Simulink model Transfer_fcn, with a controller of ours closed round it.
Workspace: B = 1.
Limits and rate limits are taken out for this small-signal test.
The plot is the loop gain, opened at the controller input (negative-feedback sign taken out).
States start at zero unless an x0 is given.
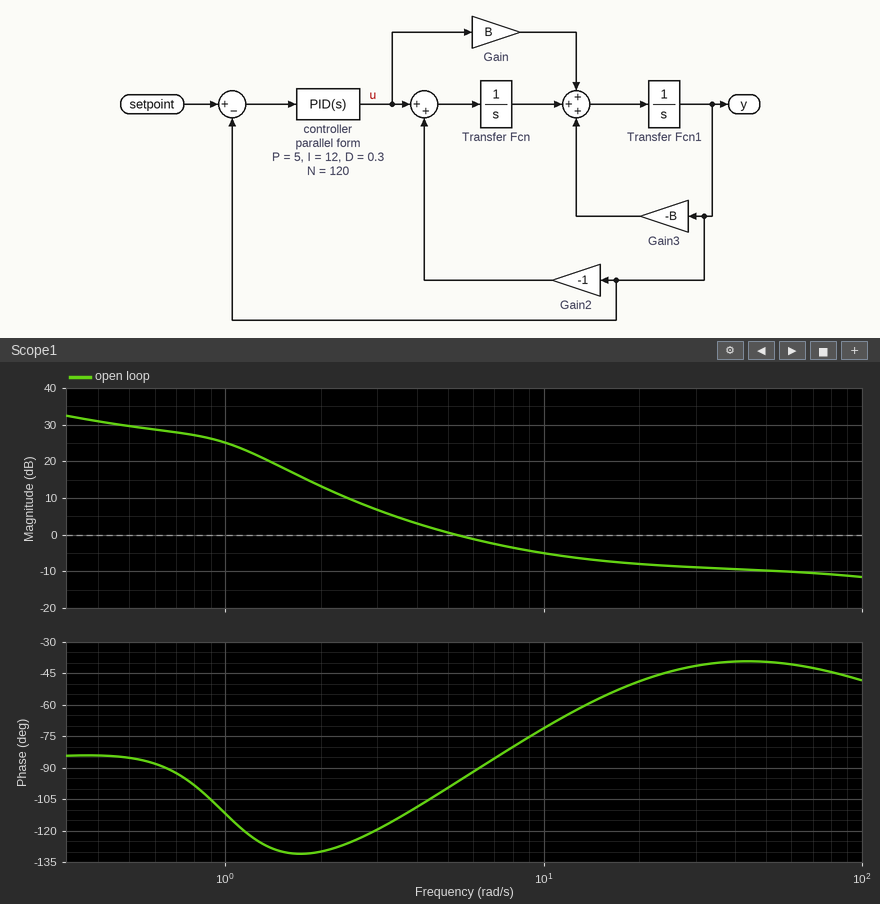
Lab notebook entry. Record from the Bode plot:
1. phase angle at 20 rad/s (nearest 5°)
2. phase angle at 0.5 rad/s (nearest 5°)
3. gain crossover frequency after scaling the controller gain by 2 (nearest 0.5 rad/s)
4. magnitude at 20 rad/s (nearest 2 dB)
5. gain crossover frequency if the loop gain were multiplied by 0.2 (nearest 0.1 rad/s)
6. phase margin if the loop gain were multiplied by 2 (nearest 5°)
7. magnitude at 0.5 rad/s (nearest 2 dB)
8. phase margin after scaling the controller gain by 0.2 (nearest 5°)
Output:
-50°
-85°
12.0 rad/s
-8 dB
1.9 rad/s
115°
30 dB
50°
